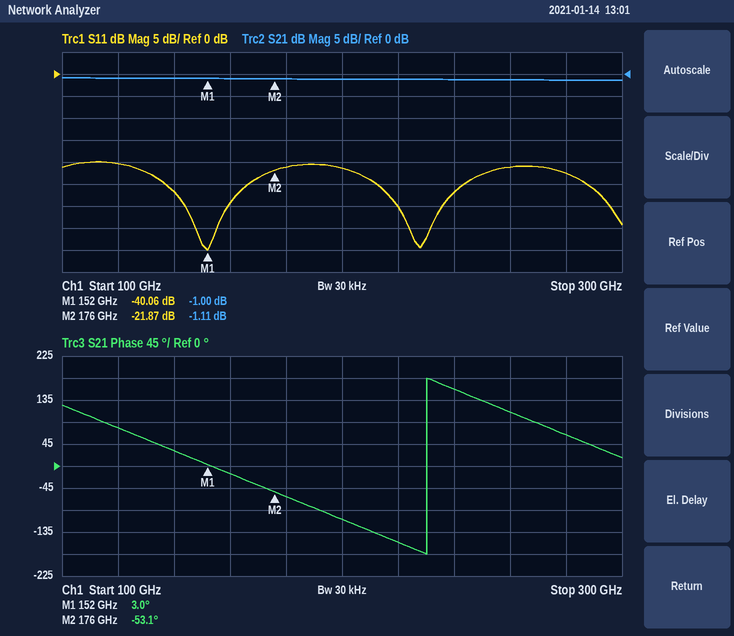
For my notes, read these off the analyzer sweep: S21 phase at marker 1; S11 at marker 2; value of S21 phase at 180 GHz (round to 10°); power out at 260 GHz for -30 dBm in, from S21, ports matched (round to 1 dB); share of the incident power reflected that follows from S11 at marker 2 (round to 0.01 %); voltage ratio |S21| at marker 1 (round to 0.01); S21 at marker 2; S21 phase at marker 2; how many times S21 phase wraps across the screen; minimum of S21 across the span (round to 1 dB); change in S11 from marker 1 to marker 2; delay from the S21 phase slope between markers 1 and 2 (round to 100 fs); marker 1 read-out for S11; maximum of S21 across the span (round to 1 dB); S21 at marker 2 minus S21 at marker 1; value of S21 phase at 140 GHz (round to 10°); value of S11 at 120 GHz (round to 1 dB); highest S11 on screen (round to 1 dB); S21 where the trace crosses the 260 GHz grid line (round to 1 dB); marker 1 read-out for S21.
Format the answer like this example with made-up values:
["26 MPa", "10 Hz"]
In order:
["3.0°", "-21.87 dB", "-60°", "-31 dBm", "0.65 %", "0.89", "-1.11 dB", "-53.1°", "1", "-1 dB", "18.19 dB", "6.5 ps", "-40.06 dB", "-1 dB", "-0.11 dB", "30°", "-20 dB", "-20 dB", "-1 dB", "-1.00 dB"]
